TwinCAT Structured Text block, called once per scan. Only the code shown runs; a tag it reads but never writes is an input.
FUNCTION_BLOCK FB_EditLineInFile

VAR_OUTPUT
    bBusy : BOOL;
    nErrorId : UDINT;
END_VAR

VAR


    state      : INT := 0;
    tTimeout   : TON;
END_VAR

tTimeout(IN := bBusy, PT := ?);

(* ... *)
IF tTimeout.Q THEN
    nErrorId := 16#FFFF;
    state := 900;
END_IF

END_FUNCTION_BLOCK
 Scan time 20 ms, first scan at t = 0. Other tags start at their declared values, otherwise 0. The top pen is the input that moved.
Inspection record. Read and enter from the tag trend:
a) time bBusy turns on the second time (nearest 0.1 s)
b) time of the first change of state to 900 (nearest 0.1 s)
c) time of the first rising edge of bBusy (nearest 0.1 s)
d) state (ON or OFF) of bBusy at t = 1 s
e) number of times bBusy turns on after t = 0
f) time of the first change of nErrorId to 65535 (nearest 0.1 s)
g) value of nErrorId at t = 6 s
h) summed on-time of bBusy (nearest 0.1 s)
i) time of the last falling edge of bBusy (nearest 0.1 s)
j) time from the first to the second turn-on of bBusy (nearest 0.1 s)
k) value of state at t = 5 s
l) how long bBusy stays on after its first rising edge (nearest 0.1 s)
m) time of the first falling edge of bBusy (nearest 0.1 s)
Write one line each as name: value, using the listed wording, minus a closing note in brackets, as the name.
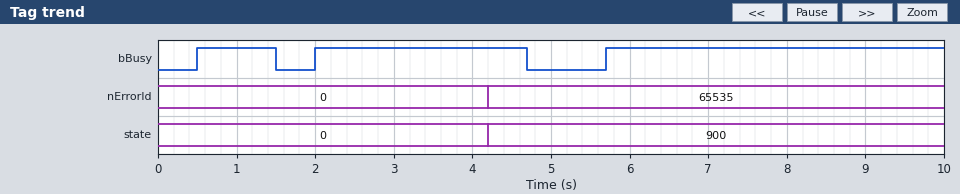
time bBusy turns on the second time: 2.0 s
time of the first change of state to 900: 4.2 s
time of the first rising edge of bBusy: 0.5 s
state (ON or OFF) of bBusy at t = 1 s: ON
number of times bBusy turns on after t = 0: 3
time of the first change of nErrorId to 65535: 4.2 s
value of nErrorId at t = 6 s: 65535
summed on-time of bBusy: 8.0 s
time of the last falling edge of bBusy: 4.7 s
time from the first to the second turn-on of bBusy: 1.5 s
value of state at t = 5 s: 900
how long bBusy stays on after its first rising edge: 1.0 s
time of the first falling edge of bBusy: 1.5 s
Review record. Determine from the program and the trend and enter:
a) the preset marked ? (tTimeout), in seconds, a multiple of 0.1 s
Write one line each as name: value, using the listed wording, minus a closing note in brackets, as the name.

the preset marked ? (tTimeout), in seconds, a multiple of 0.1 s: 2.2 s
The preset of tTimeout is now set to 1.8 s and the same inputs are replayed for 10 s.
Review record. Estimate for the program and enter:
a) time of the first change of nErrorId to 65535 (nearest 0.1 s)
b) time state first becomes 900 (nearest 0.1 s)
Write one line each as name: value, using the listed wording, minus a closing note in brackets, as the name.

time of the first change of nErrorId to 65535: 3.8 s
time state first becomes 900: 3.8 s
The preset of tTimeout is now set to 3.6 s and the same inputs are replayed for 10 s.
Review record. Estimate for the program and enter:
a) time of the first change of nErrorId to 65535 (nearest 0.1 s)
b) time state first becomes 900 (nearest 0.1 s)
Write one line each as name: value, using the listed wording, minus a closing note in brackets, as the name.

time of the first change of nErrorId to 65535: 9.3 s
time state first becomes 900: 9.3 s
